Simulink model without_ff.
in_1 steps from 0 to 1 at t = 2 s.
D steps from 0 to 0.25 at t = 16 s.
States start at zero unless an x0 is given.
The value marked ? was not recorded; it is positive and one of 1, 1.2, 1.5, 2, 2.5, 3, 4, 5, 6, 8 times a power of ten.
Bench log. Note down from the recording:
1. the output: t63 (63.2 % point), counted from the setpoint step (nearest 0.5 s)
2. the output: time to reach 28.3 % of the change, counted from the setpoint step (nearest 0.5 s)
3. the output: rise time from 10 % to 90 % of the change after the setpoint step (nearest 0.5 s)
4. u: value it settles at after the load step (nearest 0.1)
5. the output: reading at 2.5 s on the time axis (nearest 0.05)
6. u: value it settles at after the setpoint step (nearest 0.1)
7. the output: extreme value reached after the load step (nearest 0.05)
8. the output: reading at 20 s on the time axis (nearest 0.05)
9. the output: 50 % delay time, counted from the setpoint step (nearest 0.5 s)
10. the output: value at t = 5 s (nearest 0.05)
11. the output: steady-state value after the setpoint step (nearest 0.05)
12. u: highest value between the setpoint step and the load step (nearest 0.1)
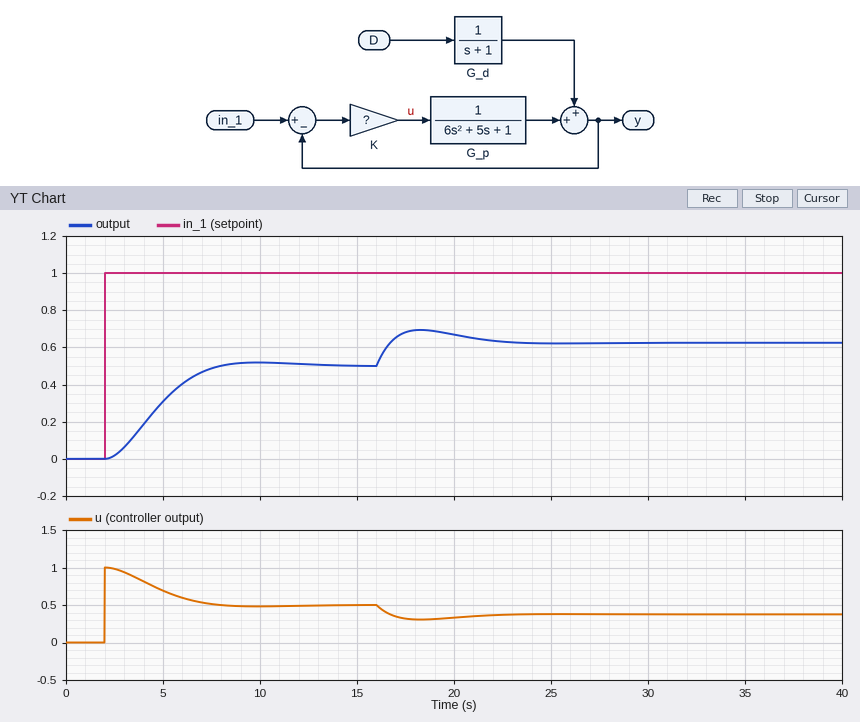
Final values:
3.0 s
1.5 s
4.0 s
0.4
0.00
0.5
0.70
0.65
2.5 s
0.30
0.50
1.0
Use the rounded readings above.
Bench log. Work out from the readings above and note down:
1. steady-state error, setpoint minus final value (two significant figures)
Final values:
0.50
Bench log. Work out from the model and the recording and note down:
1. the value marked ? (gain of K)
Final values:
1
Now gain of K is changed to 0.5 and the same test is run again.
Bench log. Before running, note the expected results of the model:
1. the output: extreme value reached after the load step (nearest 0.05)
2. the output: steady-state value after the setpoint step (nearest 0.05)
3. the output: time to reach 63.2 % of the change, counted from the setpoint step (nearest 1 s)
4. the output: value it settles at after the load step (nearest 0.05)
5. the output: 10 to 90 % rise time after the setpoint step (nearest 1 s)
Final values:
0.55
0.35
4 s
0.50
5 s
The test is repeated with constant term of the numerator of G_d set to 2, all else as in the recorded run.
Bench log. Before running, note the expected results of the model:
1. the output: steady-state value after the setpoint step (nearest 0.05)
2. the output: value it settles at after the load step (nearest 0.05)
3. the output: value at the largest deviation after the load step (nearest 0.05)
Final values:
0.50
0.75
0.90
